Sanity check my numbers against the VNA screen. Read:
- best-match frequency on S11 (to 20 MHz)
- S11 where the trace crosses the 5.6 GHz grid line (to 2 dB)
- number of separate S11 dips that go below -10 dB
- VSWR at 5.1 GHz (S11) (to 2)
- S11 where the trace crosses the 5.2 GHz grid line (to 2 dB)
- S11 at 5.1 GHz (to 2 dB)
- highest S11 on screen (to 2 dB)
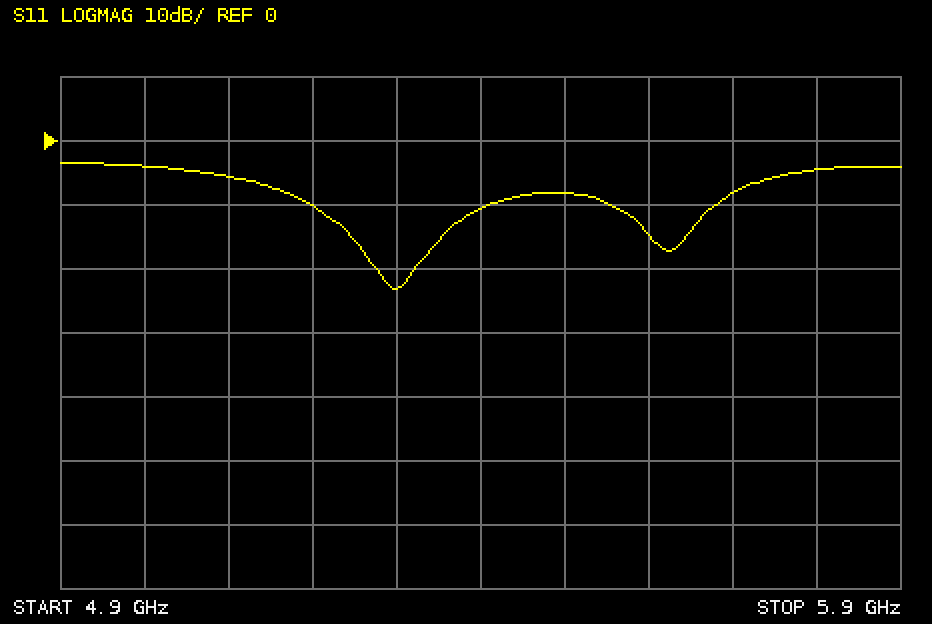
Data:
5.30 GHz
-14 dB
2
4
-10 dB
-6 dB
-4 dB
